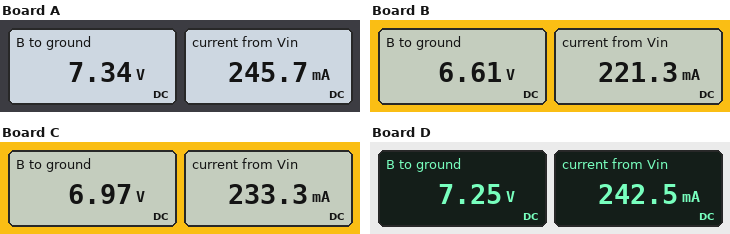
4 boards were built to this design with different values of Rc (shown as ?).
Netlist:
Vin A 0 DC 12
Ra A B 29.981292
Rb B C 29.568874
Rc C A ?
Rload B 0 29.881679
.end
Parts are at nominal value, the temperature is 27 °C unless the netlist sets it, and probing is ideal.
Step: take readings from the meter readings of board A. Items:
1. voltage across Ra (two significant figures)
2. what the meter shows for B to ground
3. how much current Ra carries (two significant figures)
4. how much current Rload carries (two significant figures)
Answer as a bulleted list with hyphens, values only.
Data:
- 4.7 V
- 7.34 V
- 160 mA
- 250 mA
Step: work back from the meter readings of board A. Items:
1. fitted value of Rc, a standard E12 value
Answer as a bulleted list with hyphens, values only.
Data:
- 22 Ω
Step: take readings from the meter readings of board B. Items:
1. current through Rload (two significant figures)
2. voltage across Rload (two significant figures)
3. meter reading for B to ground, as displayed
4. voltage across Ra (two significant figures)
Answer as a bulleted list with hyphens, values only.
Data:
- 220 mA
- 6.6 V
- 6.61 V
- 5.4 V
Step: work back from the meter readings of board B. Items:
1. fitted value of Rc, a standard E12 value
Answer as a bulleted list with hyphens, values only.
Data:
- 100 Ω
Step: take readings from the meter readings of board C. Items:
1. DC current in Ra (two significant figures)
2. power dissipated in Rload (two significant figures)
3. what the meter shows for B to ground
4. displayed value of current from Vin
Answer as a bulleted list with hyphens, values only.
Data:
- 170 mA
- 1.6 W
- 6.97 V
- 233.3 mA
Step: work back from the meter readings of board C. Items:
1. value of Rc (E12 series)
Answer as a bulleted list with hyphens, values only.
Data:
- 47 Ω
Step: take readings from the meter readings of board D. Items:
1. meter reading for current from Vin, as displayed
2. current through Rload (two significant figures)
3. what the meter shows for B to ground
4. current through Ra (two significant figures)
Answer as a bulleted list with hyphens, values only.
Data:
- 242.5 mA
- 240 mA
- 7.25 V
- 160 mA
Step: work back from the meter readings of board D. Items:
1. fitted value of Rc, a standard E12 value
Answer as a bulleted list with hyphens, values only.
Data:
- 27 Ω
